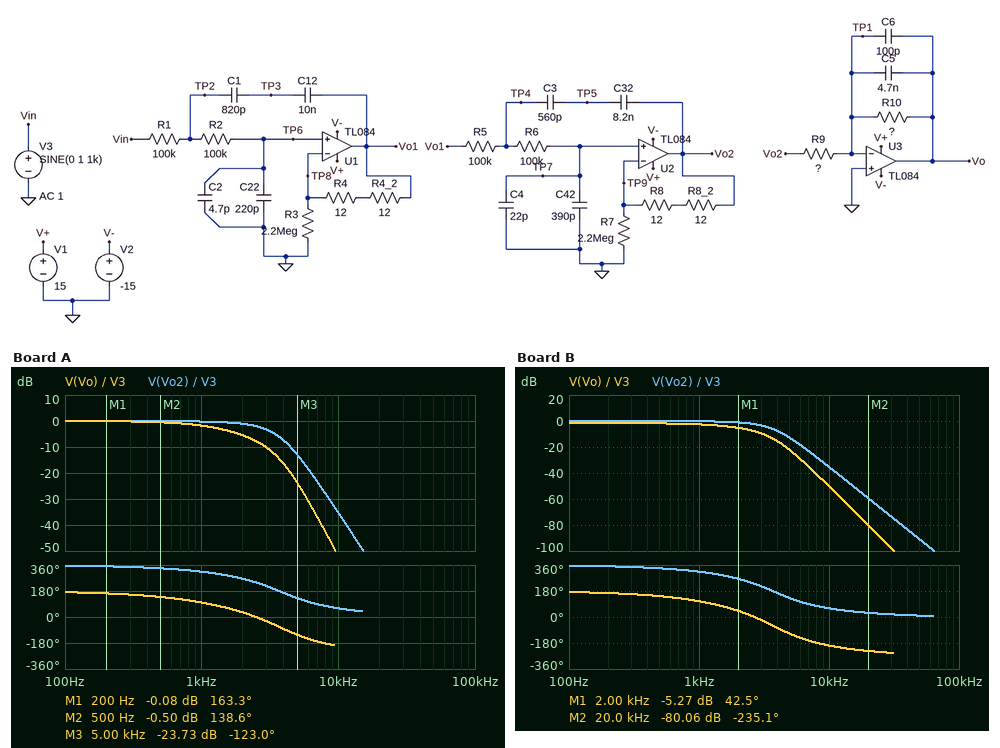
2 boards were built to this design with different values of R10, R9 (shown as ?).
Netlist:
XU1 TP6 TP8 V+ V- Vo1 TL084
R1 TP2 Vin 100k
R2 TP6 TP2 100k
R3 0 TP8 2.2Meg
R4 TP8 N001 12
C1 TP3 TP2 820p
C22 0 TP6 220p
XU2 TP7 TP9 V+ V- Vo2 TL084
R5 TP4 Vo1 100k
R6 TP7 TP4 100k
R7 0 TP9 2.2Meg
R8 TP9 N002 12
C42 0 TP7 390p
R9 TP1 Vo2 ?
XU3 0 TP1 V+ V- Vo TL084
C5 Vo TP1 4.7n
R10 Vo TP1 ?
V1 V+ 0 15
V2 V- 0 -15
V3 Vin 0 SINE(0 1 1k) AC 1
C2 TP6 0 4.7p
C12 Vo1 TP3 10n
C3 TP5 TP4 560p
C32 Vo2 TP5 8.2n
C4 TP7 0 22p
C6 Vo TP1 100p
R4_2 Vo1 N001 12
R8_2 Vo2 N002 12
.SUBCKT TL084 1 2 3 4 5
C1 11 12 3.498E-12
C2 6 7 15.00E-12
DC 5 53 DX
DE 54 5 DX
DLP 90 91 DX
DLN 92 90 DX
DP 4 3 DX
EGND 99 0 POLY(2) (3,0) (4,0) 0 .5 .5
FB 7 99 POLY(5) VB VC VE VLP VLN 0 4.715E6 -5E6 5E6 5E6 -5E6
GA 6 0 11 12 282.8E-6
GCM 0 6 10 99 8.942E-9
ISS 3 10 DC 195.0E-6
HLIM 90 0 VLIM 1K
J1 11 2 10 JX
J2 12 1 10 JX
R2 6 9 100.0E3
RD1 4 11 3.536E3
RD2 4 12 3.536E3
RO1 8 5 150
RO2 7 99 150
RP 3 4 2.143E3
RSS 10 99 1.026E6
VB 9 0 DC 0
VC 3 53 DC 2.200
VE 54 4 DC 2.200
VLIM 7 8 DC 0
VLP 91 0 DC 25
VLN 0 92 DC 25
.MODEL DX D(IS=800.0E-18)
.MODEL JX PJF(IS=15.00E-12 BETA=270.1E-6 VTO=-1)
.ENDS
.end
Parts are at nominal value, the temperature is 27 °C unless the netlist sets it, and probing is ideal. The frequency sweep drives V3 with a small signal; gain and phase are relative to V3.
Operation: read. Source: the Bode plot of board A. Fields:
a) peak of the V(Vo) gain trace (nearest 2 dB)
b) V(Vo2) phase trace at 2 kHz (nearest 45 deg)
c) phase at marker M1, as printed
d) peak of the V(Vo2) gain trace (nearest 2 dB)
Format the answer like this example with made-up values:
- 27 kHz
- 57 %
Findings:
- 0 dB
- 270 deg
- 163.3 deg
- 0 dB
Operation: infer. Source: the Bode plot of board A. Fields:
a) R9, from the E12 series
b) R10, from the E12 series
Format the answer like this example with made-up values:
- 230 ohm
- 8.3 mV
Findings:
- 22 kΩ
- 22 kΩ
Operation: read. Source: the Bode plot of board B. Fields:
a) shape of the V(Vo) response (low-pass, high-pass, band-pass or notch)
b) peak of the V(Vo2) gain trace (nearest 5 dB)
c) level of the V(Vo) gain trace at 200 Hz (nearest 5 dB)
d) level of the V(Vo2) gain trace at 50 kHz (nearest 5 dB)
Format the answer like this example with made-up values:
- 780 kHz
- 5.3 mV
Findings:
- low-pass
- 0 dB
- 0 dB
- -90 dB
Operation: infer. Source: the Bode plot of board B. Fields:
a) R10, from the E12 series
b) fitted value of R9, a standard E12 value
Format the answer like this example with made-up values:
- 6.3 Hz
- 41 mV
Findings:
- 15 kΩ
- 18 kΩ
